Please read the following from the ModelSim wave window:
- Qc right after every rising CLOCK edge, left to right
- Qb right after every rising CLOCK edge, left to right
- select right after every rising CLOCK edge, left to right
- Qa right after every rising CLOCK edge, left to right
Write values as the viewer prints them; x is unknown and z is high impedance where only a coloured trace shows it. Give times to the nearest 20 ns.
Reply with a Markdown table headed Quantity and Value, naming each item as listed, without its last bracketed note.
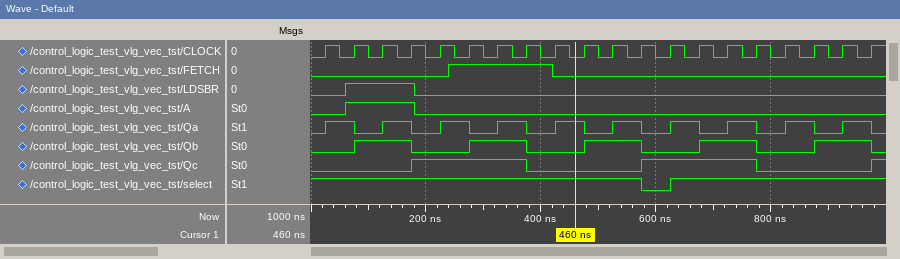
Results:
| Quantity | Value |
|---|---|
| Qc right after every rising CLOCK edge, left to right | 0 0 0 1 1 1 1 0 0 0 0 1 1 1 1 0 0 0 0 1 |
| Qb right after every rising CLOCK edge, left to right | 0 1 1 0 0 1 1 0 0 1 1 0 0 1 1 0 0 1 1 0 |
| select right after every rising CLOCK edge, left to right | 1 1 1 1 1 1 1 1 1 1 1 0 1 1 1 1 1 1 1 1 |
| Qa right after every rising CLOCK edge, left to right | 1 0 1 0 1 0 1 0 1 0 1 0 1 0 1 0 1 0 1 0 |
